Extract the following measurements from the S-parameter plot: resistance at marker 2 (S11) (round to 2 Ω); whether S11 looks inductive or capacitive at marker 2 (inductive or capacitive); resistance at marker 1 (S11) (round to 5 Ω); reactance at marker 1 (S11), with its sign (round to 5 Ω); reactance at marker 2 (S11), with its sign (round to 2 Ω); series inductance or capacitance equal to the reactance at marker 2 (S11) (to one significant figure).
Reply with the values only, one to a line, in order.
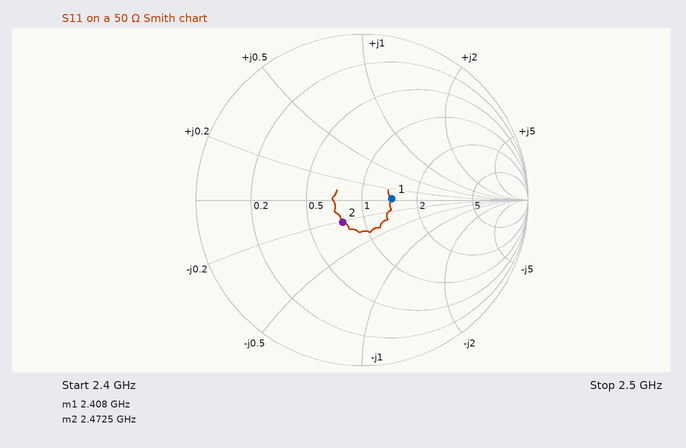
38 Ω
capacitive
70 Ω
0 Ω
-10 Ω
6 pF
